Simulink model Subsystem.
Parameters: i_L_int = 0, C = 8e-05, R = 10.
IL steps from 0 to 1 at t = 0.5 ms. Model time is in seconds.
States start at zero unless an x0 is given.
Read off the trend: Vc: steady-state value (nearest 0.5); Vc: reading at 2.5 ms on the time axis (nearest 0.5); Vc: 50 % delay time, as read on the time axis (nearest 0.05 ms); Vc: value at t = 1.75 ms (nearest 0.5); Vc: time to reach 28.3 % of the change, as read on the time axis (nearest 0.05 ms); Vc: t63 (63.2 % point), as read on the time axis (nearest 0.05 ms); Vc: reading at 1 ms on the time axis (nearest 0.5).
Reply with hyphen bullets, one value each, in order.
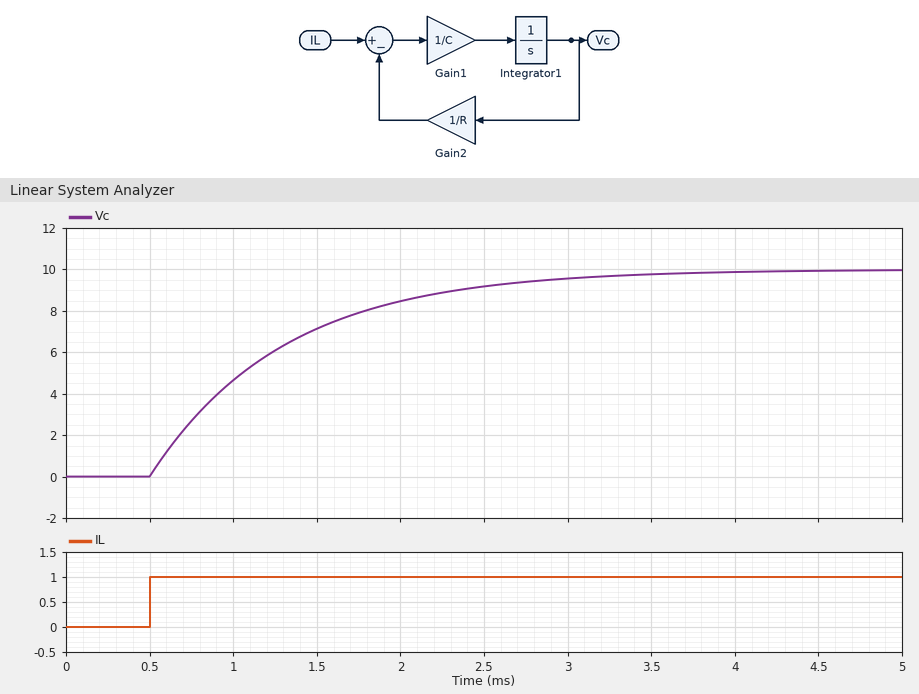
- 10.0
- 9.0
- 1.05 ms
- 8.0
- 0.75 ms
- 1.30 ms
- 4.5
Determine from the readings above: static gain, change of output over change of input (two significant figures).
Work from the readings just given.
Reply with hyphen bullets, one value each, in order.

- 10
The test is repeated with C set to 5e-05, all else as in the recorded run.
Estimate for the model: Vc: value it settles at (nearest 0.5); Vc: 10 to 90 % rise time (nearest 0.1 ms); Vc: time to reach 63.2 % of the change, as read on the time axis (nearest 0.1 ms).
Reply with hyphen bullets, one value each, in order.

- 10.0
- 1.1 ms
- 1.0 ms
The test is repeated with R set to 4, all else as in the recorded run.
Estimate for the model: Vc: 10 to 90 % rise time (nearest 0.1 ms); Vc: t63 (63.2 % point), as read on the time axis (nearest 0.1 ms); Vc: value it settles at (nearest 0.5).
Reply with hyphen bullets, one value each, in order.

- 0.7 ms
- 0.8 ms
- 4.0
